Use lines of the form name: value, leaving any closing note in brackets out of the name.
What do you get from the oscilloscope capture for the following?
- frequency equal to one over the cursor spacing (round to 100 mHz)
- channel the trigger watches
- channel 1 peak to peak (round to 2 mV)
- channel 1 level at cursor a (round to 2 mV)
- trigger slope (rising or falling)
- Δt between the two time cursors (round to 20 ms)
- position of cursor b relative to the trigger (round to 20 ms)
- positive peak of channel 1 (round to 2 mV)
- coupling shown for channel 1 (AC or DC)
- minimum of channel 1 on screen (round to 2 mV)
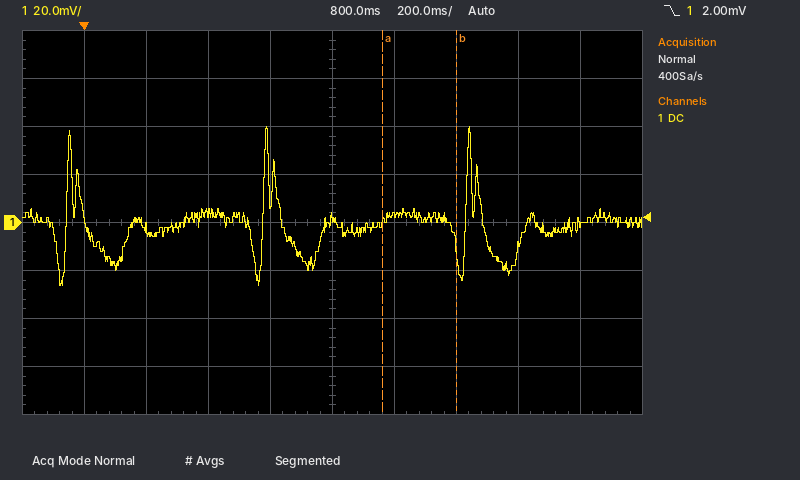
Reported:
frequency equal to one over the cursor spacing: 4.2 Hz
channel the trigger watches: channel 1
channel 1 peak to peak: 66 mV
channel 1 level at cursor a: 0 mV
trigger slope: falling
Δt between the two time cursors: 240 ms
position of cursor b relative to the trigger: +1.20 s
positive peak of channel 1: 40 mV
coupling shown for channel 1: DC
minimum of channel 1 on screen: -26 mV
